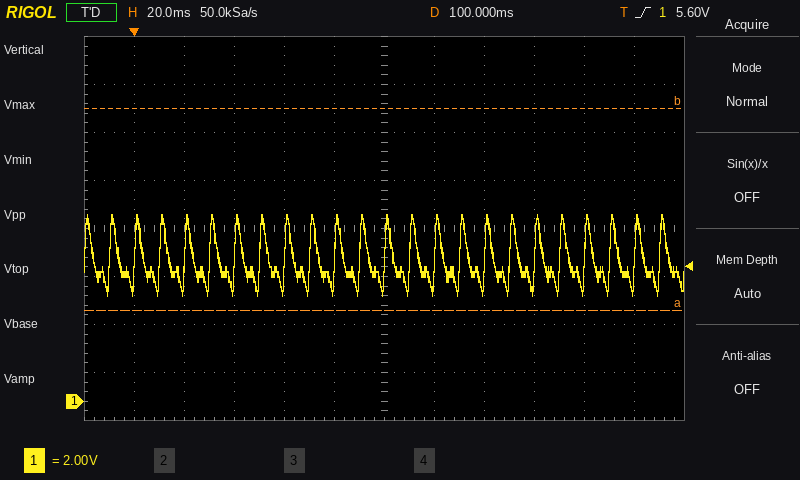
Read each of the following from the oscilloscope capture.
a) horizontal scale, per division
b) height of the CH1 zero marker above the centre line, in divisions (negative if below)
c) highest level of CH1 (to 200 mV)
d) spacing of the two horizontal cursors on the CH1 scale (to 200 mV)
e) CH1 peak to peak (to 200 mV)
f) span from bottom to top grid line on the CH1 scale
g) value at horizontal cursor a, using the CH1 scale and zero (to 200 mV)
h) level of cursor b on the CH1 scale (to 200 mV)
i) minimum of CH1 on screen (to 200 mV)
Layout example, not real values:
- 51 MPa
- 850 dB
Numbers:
- 20 ms
- -3.6 div
- 7.8 V
- 8.4 V
- 3.4 V
- 16 V
- 3.8 V
- 12.2 V
- 4.4 V
